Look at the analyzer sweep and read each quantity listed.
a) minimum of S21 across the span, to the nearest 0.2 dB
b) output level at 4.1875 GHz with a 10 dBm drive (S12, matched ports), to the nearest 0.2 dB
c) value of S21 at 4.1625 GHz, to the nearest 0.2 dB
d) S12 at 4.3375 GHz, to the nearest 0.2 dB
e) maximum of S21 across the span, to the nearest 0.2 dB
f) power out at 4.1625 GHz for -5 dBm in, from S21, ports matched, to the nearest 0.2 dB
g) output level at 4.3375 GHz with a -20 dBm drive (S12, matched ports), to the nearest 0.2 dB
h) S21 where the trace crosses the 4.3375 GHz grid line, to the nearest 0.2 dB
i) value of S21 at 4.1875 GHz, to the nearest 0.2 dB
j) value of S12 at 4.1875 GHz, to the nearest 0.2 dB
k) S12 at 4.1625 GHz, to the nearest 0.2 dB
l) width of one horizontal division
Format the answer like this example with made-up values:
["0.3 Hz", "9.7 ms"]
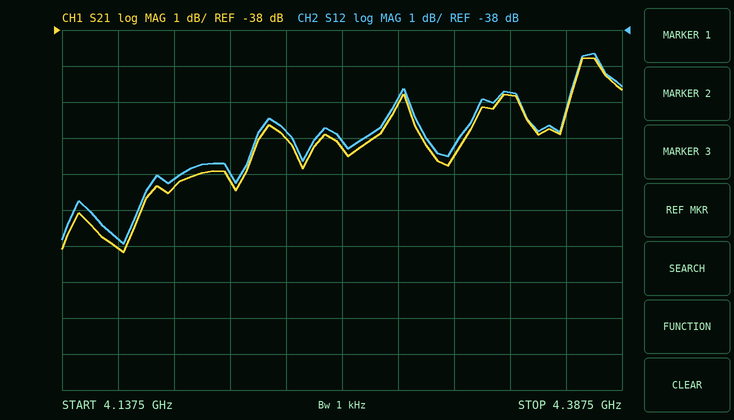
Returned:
["-44.2 dB", "-32.2 dBm", "-44.0 dB", "-39.8 dB", "-38.8 dB", "-49.0 dBm", "-59.8 dBm", "-39.8 dB", "-42.4 dB", "-42.2 dB", "-43.8 dB", "25 MHz"]
